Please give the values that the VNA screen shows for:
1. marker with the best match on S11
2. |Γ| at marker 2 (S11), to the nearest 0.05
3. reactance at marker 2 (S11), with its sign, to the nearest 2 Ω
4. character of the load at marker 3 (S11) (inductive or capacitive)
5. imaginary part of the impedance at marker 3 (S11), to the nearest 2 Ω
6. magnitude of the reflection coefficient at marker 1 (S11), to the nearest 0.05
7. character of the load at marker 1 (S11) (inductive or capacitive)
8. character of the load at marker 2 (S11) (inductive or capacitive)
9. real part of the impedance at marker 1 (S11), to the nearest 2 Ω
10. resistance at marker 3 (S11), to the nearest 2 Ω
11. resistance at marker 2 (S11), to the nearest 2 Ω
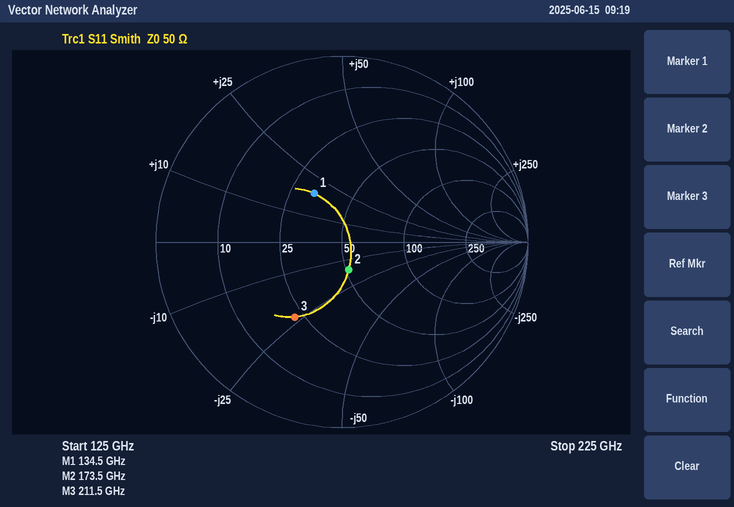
marker 2
0.15
-16 Ω
capacitive
-24 Ω
0.30
inductive
capacitive
32 Ω
22 Ω
52 Ω
